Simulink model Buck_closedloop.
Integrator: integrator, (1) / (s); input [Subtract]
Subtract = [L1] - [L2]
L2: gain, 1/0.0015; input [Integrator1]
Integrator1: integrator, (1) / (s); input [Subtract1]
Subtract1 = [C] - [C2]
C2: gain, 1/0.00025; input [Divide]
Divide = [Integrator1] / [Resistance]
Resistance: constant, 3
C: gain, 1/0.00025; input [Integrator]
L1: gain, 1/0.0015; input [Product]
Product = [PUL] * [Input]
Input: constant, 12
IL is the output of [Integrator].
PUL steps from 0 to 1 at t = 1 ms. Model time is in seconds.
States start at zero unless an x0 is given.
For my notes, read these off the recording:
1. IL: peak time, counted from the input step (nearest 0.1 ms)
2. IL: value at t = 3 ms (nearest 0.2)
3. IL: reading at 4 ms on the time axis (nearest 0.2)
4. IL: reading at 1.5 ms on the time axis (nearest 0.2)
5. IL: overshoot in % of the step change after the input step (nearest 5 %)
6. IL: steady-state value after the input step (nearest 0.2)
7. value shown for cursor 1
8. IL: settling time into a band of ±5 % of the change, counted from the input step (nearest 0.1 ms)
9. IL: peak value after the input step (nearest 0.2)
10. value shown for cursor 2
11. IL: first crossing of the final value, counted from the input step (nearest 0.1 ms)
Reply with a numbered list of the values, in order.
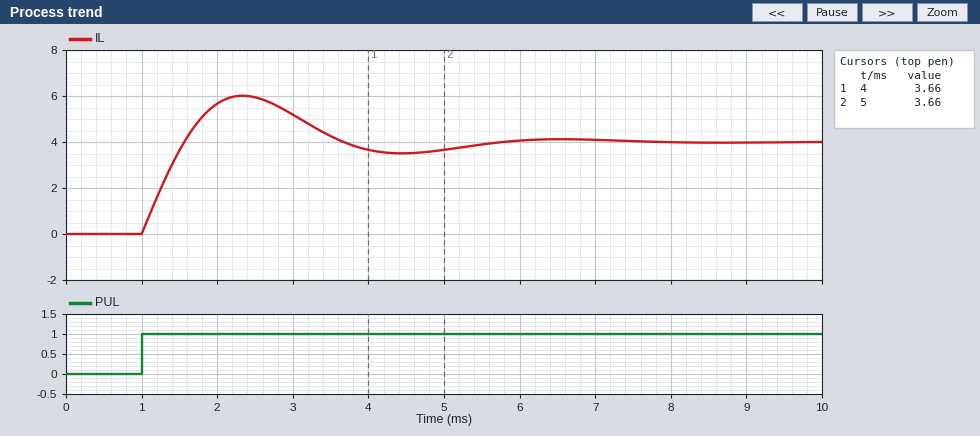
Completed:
1. 1.3 ms
2. 5.2
3. 3.6
4. 3.6
5. 50 %
6. 4.0
7. 3.66
8. 4.3 ms
9. 6.0
10. 3.66
11. 0.6 ms
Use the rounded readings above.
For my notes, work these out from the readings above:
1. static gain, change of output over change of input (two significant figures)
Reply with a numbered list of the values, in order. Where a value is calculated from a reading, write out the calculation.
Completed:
1. (4 - 0) / (1 - 0) = 4.0
